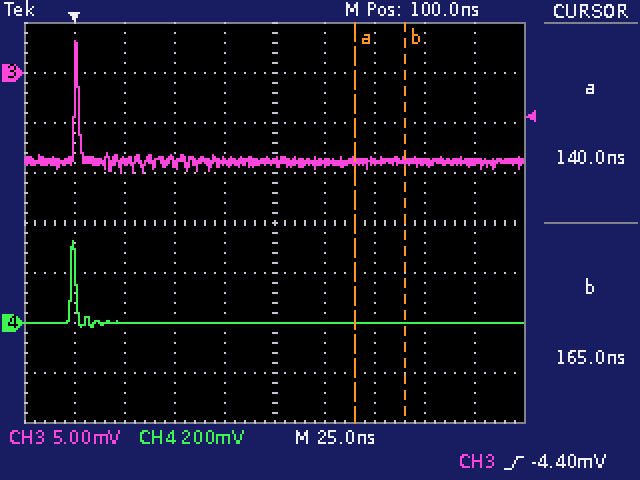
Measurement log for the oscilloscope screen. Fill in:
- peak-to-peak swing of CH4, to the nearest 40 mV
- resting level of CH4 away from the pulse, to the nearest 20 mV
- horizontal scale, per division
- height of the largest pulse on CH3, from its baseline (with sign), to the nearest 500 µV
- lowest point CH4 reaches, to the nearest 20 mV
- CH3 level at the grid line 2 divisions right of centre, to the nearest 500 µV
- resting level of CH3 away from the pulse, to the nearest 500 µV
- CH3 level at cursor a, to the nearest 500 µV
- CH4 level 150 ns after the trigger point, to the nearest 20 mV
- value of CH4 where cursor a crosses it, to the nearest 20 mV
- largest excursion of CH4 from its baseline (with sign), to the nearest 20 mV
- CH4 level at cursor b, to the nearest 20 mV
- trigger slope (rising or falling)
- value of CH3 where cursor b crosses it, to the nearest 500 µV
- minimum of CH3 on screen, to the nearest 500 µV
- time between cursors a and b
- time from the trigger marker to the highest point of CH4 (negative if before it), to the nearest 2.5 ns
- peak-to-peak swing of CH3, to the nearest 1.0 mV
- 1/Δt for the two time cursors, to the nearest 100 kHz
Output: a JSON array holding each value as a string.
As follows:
["360 mV", "0 mV", "25 ns", "+12.0 mV", "-20 mV", "-9.0 mV", "-9.0 mV", "-9.0 mV", "0 mV", "0 mV", "+320 mV", "0 mV", "rising", "-9.0 mV", "-10.0 mV", "25.0 ns", "0.0 ns", "13.0 mV", "40.0 MHz"]
